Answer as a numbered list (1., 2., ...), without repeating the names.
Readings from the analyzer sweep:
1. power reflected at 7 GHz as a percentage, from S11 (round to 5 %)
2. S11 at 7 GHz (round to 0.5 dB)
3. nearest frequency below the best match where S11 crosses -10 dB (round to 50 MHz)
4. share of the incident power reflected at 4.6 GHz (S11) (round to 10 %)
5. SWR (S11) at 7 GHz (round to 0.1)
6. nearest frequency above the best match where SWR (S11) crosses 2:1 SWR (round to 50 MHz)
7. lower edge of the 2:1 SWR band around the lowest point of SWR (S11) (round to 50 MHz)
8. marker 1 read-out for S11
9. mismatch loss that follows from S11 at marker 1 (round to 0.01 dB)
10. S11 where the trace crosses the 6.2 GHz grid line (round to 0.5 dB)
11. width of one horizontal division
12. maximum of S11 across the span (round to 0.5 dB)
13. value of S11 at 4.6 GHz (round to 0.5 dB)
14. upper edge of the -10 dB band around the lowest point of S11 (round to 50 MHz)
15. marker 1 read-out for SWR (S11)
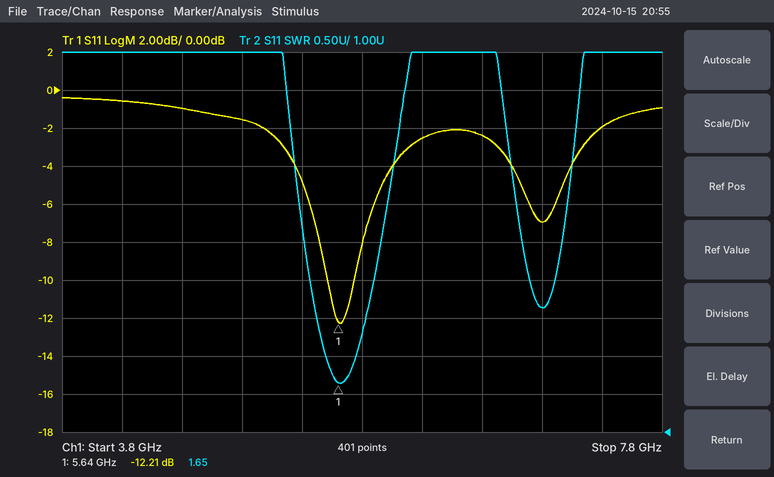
1. 20 %
2. -7.0 dB
3. 5.55 GHz
4. 80 %
5. 2.6
6. 5.75 GHz
7. 5.55 GHz
8. -12.21 dB
9. 0.27 dB
10. -2.5 dB
11. 400 MHz
12. -0.5 dB
13. -1.0 dB
14. 5.75 GHz
15. 1.65
